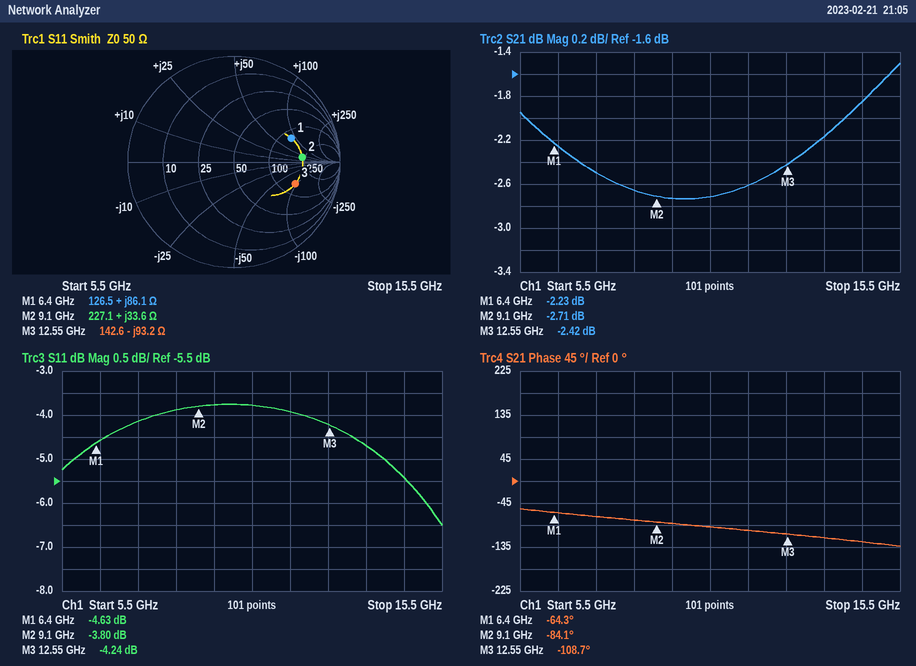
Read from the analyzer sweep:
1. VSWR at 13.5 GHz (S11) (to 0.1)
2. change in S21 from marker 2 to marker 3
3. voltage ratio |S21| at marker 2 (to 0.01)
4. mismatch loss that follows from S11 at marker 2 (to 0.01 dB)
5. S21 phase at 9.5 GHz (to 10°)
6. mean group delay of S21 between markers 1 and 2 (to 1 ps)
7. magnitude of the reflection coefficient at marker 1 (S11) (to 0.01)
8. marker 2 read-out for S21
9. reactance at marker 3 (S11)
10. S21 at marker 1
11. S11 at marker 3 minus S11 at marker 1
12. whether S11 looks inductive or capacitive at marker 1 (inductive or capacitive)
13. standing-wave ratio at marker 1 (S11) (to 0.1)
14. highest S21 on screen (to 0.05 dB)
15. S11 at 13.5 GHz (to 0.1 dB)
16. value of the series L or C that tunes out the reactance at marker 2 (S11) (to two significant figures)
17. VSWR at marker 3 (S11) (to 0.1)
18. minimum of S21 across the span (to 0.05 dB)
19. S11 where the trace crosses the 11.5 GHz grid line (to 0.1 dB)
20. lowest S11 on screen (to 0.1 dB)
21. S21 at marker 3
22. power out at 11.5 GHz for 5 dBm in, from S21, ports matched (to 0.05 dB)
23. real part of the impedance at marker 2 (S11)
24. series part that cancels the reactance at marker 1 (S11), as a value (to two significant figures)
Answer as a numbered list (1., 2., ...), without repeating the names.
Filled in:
1. 3.8
2. 0.29 dB
3. 0.73
4. 2.34 dB
5. -90°
6. 20 ps
7. 0.59
8. -2.71 dB
9. -93.2 Ω
10. -2.23 dB
11. 0.39 dB
12. inductive
13. 3.8
14. -1.50 dB
15. -4.7 dB
16. 520 fF
17. 4.2
18. -2.75 dB
19. -3.9 dB
20. -6.5 dB
21. -2.42 dB
22. 2.40 dBm
23. 227.1 Ω
24. 290 fF
